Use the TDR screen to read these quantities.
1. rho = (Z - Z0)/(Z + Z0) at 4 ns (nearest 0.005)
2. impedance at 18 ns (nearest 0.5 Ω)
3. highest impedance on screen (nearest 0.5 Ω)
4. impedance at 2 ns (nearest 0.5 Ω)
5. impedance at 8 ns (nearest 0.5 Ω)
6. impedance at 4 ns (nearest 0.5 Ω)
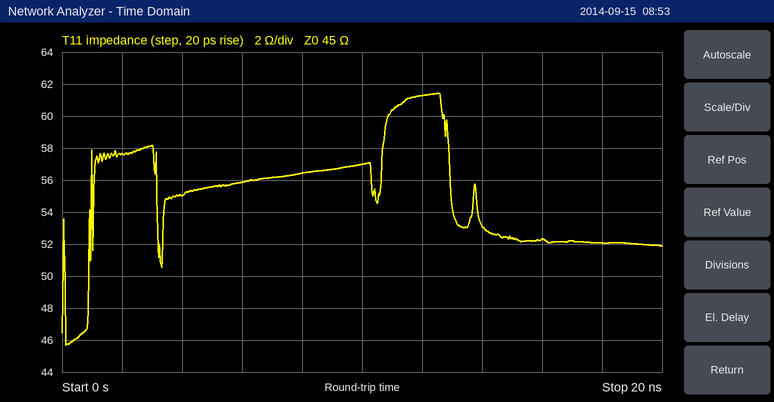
+0.100
52.0 Ω
61.5 Ω
57.5 Ω
56.5 Ω
55.0 Ω
